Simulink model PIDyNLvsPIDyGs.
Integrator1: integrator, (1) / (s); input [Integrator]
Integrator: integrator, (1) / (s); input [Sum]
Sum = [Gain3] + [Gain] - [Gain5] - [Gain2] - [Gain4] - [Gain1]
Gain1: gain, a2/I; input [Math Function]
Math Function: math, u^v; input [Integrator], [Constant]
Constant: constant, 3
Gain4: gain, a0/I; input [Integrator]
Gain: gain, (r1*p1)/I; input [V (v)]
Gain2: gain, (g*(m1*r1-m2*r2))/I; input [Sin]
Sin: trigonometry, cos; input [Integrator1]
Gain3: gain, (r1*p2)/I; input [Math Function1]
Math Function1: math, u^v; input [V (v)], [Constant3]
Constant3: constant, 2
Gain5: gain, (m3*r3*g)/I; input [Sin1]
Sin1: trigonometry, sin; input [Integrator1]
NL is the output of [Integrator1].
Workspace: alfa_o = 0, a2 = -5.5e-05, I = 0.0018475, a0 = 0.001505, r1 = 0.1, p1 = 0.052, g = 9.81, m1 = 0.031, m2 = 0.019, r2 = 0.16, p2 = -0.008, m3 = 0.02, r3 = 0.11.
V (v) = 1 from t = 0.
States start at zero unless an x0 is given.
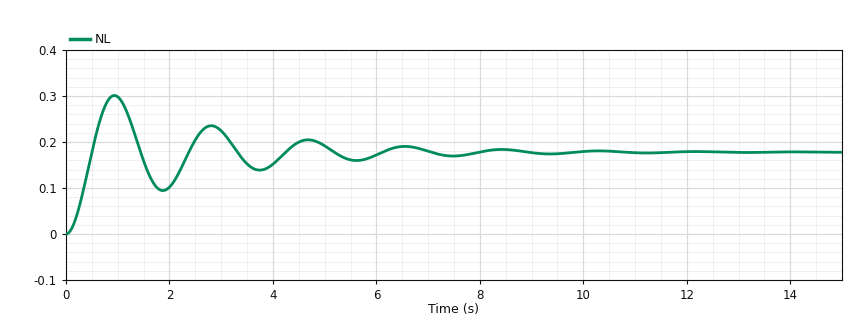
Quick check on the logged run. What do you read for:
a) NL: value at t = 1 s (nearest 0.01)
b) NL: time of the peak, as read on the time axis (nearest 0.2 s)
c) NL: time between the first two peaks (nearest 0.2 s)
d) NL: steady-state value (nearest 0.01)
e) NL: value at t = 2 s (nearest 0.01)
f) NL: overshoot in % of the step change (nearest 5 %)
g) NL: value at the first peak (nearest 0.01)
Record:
0.30
1.0 s
1.8 s
0.18
0.10
70 %
0.30
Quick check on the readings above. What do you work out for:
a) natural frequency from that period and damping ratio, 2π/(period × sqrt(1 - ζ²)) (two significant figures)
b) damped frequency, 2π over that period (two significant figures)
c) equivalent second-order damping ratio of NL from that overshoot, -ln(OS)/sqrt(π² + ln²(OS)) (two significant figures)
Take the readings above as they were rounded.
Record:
3.5 rad/s
3.5 rad/s
0.11
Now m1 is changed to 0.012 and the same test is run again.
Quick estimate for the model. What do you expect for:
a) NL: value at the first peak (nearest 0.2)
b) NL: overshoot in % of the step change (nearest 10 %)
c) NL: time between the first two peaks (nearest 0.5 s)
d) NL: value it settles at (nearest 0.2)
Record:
1.6
80 %
1.5 s
0.8
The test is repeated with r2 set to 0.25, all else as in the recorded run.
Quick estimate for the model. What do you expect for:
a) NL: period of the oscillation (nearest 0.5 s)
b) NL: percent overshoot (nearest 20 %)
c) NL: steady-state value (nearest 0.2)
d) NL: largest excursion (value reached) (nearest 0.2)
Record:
1.5 s
80 %
0.8
1.4
